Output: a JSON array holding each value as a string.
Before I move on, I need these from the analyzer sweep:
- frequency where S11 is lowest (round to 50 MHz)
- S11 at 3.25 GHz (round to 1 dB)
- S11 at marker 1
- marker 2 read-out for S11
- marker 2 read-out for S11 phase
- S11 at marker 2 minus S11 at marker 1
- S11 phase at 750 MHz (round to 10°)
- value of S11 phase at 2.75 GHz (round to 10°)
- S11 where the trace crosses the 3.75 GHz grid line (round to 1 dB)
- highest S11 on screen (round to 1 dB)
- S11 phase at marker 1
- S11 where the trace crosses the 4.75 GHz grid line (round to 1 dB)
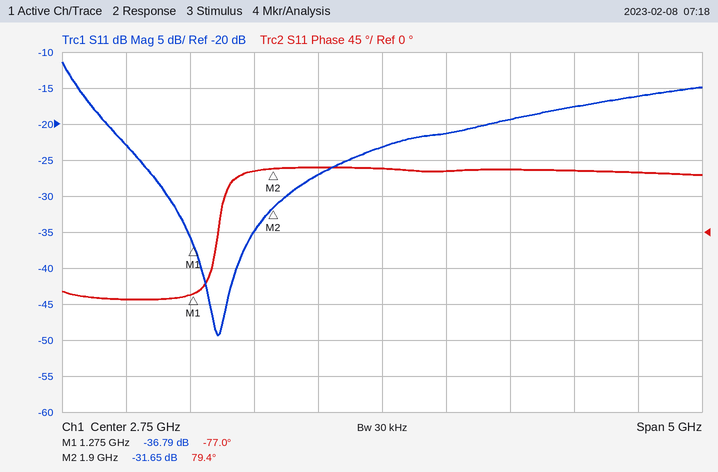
["1.45 GHz", "-21 dB", "-36.79 dB", "-31.65 dB", "79.4°", "5.14 dB", "-80°", "80°", "-19 dB", "-11 dB", "-77.0°", "-16 dB"]
